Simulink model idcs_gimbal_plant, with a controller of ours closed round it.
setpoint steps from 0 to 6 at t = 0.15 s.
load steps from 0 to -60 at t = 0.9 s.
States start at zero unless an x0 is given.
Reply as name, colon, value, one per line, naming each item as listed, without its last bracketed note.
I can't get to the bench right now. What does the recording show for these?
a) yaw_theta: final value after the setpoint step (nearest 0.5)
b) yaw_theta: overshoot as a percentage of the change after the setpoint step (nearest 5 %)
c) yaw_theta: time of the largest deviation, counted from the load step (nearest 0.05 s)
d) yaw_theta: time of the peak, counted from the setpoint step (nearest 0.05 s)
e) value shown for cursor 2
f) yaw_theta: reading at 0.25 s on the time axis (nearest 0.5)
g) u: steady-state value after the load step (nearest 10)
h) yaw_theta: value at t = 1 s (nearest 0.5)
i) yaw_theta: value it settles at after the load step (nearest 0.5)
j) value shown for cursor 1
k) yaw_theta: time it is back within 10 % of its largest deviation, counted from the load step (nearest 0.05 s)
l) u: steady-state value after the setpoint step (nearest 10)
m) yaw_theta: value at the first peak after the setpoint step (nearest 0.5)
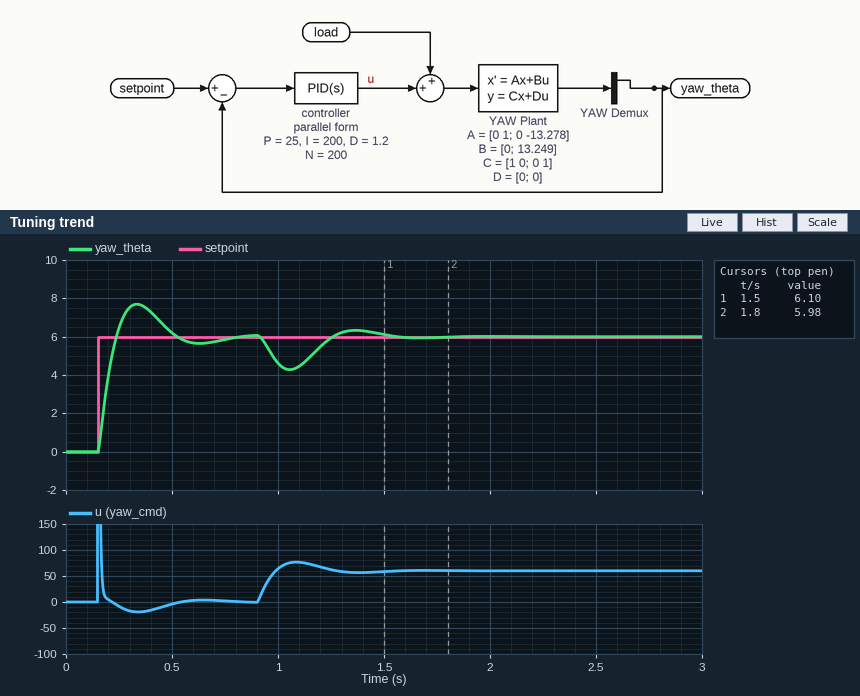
yaw_theta: final value after the setpoint step: 6.0
yaw_theta: overshoot as a percentage of the change after the setpoint step: 30 %
yaw_theta: time of the largest deviation, counted from the load step: 0.15 s
yaw_theta: time of the peak, counted from the setpoint step: 0.20 s
value shown for cursor 2: 5.98
yaw_theta: reading at 0.25 s on the time axis: 6.5
u: steady-state value after the load step: 60
yaw_theta: value at t = 1 s: 4.5
yaw_theta: value it settles at after the load step: 6.0
value shown for cursor 1: 6.10
yaw_theta: time it is back within 10 % of its largest deviation, counted from the load step: 0.55 s
u: steady-state value after the setpoint step: 0
yaw_theta: value at the first peak after the setpoint step: 7.5
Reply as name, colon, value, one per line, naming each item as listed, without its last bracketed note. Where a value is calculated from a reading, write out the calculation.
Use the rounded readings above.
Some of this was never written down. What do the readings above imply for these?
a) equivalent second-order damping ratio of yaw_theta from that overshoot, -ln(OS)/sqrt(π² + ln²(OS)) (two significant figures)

equivalent second-order damping ratio of yaw_theta from that overshoot, -ln(OS)/sqrt(π² + ln²(OS)): ln(0.3) = -1.204; 1.204 / sqrt(9.870 + 1.450) = 0.36
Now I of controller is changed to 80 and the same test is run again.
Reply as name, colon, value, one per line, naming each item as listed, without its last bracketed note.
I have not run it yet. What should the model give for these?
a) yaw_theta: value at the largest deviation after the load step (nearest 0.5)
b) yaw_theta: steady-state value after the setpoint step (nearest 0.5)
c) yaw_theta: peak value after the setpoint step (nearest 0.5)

yaw_theta: value at the largest deviation after the load step: 4.0
yaw_theta: steady-state value after the setpoint step: 6.0
yaw_theta: peak value after the setpoint step: 7.0
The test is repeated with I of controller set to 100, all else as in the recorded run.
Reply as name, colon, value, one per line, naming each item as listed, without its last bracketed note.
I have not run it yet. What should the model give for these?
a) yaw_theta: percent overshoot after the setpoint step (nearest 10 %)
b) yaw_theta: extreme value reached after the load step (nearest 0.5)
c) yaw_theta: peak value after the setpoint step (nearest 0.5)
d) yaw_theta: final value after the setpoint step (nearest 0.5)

yaw_theta: percent overshoot after the setpoint step: 20 %
yaw_theta: extreme value reached after the load step: 4.0
yaw_theta: peak value after the setpoint step: 7.0
yaw_theta: final value after the setpoint step: 6.0
